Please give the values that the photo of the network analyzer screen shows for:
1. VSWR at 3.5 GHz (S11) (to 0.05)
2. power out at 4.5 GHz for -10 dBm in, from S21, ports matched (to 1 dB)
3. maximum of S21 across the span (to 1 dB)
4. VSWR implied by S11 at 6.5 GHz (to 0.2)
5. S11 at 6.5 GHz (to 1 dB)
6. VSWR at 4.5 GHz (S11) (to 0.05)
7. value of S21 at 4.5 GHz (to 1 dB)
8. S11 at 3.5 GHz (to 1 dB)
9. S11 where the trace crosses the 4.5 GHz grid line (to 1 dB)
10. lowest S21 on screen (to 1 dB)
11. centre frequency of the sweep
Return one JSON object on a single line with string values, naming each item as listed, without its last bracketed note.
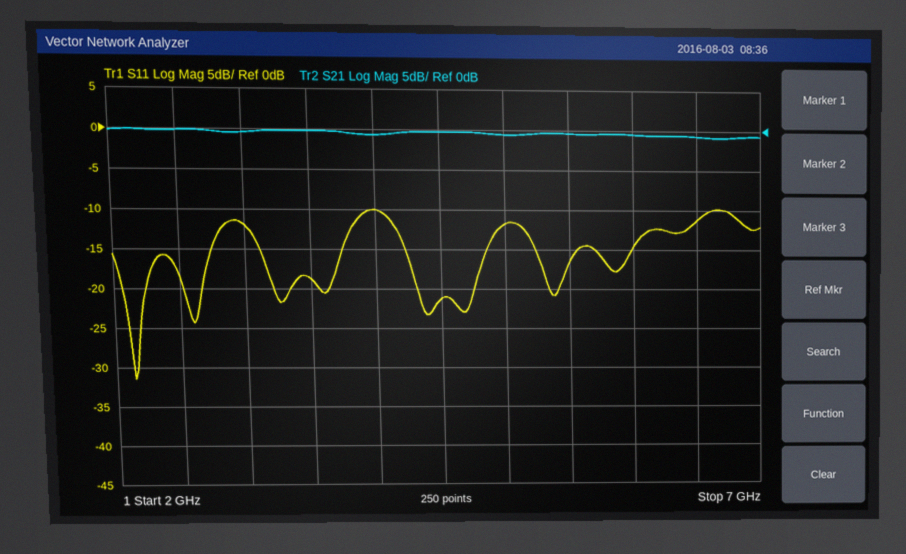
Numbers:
{"VSWR at 3.5 GHz (S11)": "1.25", "power out at 4.5 GHz for -10 dBm in, from S21, ports matched": "-10 dBm", "maximum of S21 across the span": "0 dB", "VSWR implied by S11 at 6.5 GHz": "1.8", "S11 at 6.5 GHz": "-11 dB", "VSWR at 4.5 GHz (S11)": "1.20", "value of S21 at 4.5 GHz": "0 dB", "S11 at 3.5 GHz": "-19 dB", "S11 where the trace crosses the 4.5 GHz grid line": "-21 dB", "lowest S21 on screen": "-1 dB", "centre frequency of the sweep": "4.5 GHz"}
